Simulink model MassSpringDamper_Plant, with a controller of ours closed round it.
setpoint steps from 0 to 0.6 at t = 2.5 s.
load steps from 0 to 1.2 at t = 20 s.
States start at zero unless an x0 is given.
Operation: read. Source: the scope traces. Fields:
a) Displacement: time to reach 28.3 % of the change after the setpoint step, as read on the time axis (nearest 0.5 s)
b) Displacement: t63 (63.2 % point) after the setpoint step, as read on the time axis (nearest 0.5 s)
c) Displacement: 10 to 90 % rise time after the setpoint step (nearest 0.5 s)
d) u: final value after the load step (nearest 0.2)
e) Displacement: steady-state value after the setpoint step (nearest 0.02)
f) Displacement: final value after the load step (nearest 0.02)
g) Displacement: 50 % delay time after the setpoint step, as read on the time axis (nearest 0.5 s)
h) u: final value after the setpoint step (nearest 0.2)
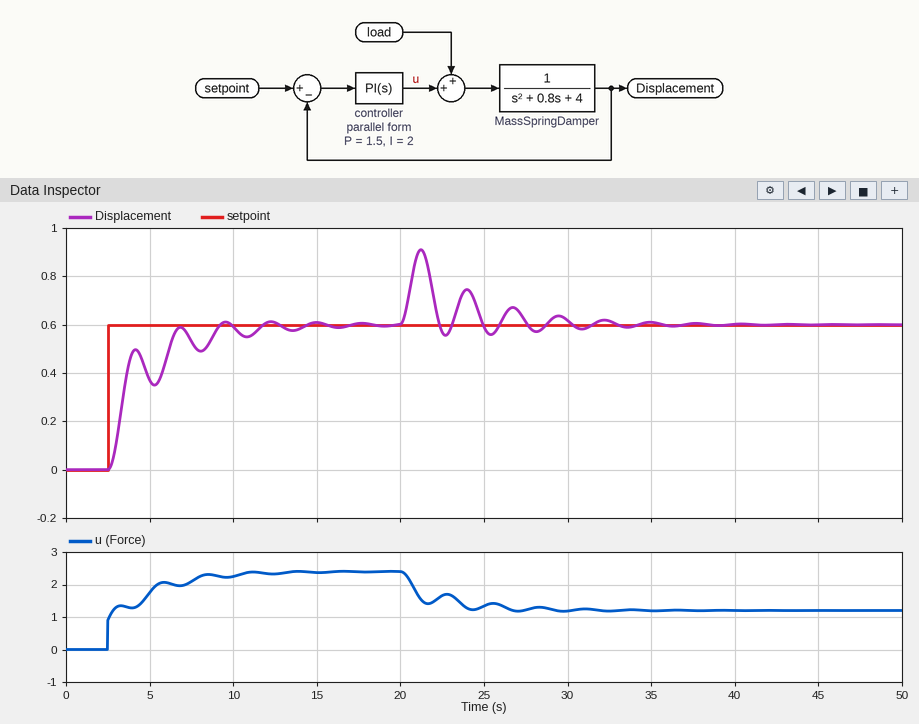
3.0 s
3.5 s
3.5 s
1.2
0.60
0.60
3.5 s
2.4
